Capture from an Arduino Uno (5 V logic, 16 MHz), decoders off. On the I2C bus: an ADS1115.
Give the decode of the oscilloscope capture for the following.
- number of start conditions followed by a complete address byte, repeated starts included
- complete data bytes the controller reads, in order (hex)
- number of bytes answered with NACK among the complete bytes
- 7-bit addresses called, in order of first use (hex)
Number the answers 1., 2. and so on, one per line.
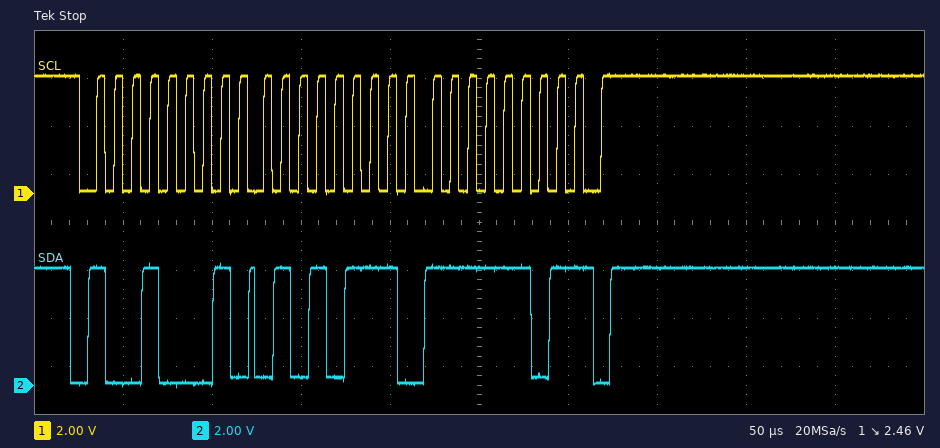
1. 1
2. 57 FD
3. 1
4. 0x48
